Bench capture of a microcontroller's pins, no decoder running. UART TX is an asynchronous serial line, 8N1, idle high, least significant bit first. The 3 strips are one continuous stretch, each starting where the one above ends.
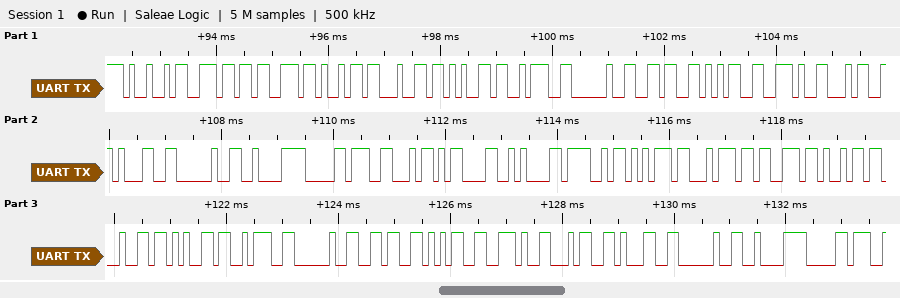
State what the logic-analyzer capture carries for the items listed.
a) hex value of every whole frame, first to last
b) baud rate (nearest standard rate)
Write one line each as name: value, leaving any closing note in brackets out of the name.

hex value of every whole frame, first to last: 0x49 0x6E 0x73 0x69 0x64 0x65 0x3A 0x20 0x36 0x35 0x2E 0x34 0x31 0x20 0xC2 0xB0 0x46 0x0D 0x0A 0x4F 0x75 0x74 0x73 0x69 0x64 0x65 0x3A 0x20 0x36 0x35 0x2E 0x34 0x31 0x20 0xC2 0xB0
baud rate: 9600 baud
